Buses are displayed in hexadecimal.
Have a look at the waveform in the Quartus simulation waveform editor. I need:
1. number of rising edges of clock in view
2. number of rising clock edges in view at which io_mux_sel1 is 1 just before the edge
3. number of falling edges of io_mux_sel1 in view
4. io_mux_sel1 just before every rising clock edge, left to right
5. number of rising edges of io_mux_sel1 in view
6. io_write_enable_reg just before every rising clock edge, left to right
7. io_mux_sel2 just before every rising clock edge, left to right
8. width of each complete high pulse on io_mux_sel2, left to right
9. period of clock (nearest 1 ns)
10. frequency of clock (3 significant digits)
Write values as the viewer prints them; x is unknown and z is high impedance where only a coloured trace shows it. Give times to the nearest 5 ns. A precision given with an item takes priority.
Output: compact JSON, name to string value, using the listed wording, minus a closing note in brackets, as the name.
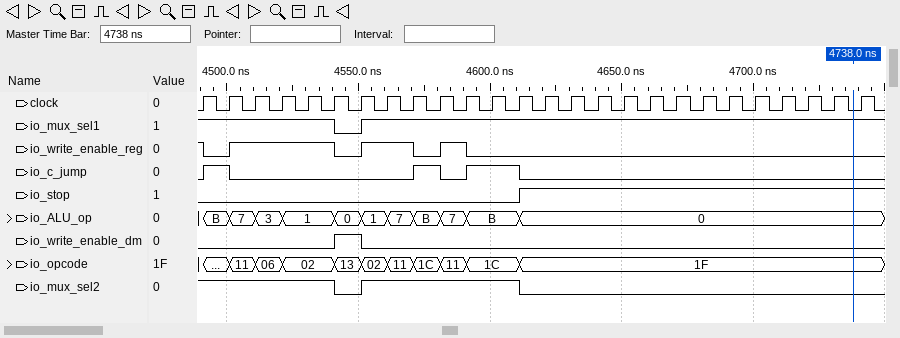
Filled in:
{"number of rising edges of clock in view": "26", "number of rising clock edges in view at which io_mux_sel1 is 1 just before the edge": "25", "number of falling edges of io_mux_sel1 in view": "1", "io_mux_sel1 just before every rising clock edge, left to right": "1 1 1 1 1 1 0 1 1 1 1 1 1 1 1 1 1 1 1 1 1 1 1 1 1 1", "number of rising edges of io_mux_sel1 in view": "1", "io_write_enable_reg just before every rising clock edge, left to right": "1 0 1 1 1 1 0 1 1 0 1 0 0 0 0 0 0 0 0 0 0 0 0 0 0 0", "io_mux_sel2 just before every rising clock edge, left to right": "1 1 1 1 1 1 0 1 1 1 1 1 1 0 0 0 0 0 0 0 0 0 0 0 0 0", "width of each complete high pulse on io_mux_sel2, left to right": "60 ns", "period of clock": "10 ns", "frequency of clock": "100 MHz"}
